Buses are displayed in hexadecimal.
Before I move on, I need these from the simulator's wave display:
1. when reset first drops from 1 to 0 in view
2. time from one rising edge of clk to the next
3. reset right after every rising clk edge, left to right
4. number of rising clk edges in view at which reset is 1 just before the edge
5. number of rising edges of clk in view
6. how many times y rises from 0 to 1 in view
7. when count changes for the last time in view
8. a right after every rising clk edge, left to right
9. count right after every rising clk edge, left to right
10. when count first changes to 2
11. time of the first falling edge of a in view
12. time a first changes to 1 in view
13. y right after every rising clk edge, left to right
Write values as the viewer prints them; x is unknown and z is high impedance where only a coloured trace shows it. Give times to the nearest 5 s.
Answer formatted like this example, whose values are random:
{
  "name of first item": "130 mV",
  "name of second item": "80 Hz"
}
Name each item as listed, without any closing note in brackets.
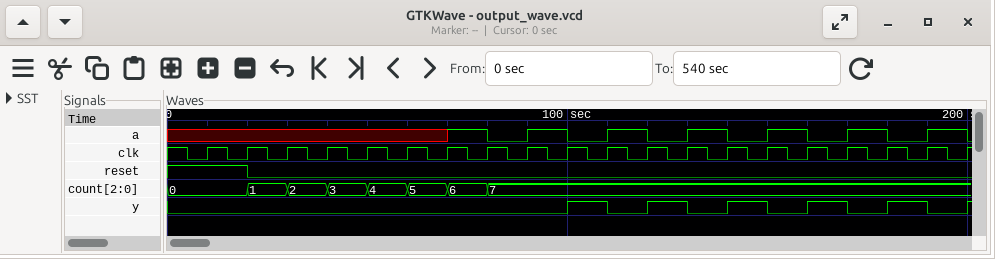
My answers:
{
  "when reset first drops from 1 to 0 in view": "20 s",
  "time from one rising edge of clk to the next": "10 s",
  "reset right after every rising clk edge, left to right": "1 0 0 0 0 0 0 0 0 0 0 0 0 0 0 0 0 0 0 0",
  "number of rising clk edges in view at which reset is 1 just before the edge": "2",
  "number of rising edges of clk in view": "20",
  "how many times y rises from 0 to 1 in view": "6",
  "when count changes for the last time in view": "80 s",
  "a right after every rising clk edge, left to right": "x x x x x x 1 0 1 0 1 0 1 0 1 0 1 0 1 0",
  "count right after every rising clk edge, left to right": "0, 1, 2, 3, 4, 5, 6, 7, 7, 7, 7, 7, 7, 7, 7, 7, 7, 7, 7, 7",
  "when count first changes to 2": "30 s",
  "time of the first falling edge of a in view": "80 s",
  "time a first changes to 1 in view": "70 s",
  "y right after every rising clk edge, left to right": "0 0 0 0 0 0 0 0 0 1 0 1 0 1 0 1 0 1 0 1"
}
